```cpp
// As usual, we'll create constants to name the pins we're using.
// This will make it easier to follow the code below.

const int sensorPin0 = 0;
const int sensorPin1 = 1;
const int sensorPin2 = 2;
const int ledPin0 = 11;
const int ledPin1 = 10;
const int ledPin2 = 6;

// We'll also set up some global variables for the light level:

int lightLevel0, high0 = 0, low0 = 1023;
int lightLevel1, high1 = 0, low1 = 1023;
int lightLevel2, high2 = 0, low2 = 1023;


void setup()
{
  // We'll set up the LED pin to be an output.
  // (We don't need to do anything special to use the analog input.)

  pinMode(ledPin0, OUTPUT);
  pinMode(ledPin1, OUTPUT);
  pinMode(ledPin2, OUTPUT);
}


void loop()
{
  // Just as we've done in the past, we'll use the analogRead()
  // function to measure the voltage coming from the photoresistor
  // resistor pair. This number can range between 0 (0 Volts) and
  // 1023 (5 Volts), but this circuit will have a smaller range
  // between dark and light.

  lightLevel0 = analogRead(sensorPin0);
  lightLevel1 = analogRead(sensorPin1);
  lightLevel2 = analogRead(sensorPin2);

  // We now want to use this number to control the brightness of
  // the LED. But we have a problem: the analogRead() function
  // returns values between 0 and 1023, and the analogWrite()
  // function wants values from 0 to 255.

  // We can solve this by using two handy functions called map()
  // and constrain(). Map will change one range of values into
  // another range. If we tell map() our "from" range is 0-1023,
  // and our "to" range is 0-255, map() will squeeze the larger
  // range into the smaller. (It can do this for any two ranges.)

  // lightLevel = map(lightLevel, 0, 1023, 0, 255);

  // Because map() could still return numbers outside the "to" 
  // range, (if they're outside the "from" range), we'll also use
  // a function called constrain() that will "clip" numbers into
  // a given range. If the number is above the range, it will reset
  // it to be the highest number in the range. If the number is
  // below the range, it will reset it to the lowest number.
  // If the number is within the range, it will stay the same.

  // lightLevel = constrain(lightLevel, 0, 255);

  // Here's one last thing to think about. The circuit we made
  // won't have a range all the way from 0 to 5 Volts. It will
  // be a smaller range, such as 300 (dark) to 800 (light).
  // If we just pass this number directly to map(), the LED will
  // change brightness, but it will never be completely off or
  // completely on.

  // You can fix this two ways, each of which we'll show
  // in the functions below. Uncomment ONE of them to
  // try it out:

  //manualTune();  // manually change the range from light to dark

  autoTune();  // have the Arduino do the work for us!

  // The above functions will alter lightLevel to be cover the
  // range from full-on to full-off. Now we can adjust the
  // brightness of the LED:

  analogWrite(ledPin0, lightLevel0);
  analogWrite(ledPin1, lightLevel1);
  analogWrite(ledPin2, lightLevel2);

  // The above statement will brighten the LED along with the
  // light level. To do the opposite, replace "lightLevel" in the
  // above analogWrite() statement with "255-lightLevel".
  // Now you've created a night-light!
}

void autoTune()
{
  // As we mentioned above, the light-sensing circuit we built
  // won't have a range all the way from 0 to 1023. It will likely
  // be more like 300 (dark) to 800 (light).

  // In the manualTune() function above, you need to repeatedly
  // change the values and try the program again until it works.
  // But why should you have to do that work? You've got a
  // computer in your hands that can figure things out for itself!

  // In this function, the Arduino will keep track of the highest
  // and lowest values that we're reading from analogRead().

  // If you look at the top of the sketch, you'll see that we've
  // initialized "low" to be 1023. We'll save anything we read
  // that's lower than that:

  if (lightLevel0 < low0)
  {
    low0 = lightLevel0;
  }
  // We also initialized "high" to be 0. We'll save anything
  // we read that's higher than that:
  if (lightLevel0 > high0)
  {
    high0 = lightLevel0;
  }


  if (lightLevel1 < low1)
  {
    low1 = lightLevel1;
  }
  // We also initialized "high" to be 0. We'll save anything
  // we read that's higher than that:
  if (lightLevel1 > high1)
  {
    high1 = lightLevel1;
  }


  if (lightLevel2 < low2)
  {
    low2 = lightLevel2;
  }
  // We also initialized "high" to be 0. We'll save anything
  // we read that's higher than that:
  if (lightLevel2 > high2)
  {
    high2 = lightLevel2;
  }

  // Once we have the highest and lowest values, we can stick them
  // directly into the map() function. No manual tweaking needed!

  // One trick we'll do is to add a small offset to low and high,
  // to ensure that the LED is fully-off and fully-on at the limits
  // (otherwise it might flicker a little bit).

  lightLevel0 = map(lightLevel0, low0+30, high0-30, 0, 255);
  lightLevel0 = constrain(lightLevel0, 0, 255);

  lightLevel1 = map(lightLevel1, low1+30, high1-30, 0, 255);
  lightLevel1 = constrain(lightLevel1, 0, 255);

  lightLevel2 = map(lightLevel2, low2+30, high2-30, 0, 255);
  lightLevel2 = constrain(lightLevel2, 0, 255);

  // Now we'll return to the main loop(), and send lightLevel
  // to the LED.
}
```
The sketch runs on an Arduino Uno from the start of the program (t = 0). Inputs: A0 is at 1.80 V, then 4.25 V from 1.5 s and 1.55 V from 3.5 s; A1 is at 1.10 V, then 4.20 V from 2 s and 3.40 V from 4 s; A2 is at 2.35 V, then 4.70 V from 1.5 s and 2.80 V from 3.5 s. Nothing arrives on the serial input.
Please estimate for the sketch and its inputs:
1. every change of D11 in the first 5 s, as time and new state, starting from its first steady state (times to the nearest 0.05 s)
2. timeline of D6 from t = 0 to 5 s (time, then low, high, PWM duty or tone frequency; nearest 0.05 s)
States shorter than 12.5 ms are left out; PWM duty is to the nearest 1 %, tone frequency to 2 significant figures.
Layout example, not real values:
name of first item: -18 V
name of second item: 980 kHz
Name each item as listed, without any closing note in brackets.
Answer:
every change of D11 in the first 5 s, as time and new state, starting from its first steady state: 0 s PWM 50 %; 1.5 s high; 3.5 s low
timeline of D6 from t = 0 to 5 s: 0 s PWM 50 %; 1.5 s high; 3.5 s PWM 15 %
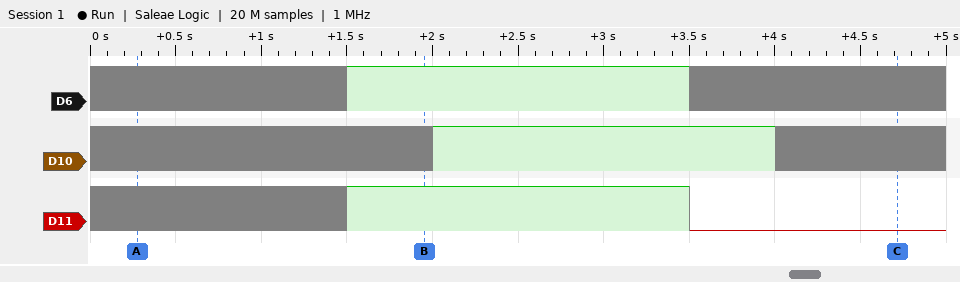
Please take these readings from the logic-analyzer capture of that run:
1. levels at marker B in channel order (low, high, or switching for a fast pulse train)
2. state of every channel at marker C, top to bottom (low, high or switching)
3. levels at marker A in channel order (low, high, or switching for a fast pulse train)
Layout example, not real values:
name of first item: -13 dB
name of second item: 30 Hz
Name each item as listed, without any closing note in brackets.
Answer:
levels at marker B in channel order: D6 high, D10 switching, D11 high
state of every channel at marker C, top to bottom: D6 switching, D10 switching, D11 low
levels at marker A in channel order: D6 switching, D10 switching, D11 switching
